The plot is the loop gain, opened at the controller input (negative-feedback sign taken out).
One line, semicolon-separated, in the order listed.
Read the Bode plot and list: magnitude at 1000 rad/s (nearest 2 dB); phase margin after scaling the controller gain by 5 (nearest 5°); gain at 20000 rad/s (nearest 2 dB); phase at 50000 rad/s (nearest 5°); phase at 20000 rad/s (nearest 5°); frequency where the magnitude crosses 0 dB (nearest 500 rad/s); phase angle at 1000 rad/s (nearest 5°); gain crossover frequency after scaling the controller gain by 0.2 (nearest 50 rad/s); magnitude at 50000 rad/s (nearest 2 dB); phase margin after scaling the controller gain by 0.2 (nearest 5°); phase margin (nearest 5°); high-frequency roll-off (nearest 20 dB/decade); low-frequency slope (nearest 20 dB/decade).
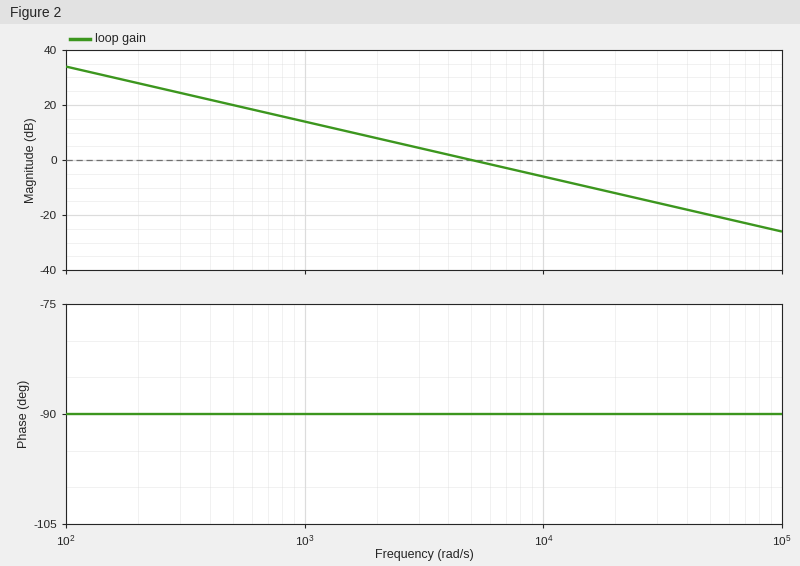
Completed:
14 dB; 90°; -12 dB; -90°; -90°; 5000 rad/s; -90°; 1000 rad/s; -20 dB; 90°; 90°; -20 dB/decade; -20 dB/decade
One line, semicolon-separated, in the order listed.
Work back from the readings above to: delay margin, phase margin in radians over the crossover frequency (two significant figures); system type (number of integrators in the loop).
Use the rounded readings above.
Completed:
0.00031 s; 1
